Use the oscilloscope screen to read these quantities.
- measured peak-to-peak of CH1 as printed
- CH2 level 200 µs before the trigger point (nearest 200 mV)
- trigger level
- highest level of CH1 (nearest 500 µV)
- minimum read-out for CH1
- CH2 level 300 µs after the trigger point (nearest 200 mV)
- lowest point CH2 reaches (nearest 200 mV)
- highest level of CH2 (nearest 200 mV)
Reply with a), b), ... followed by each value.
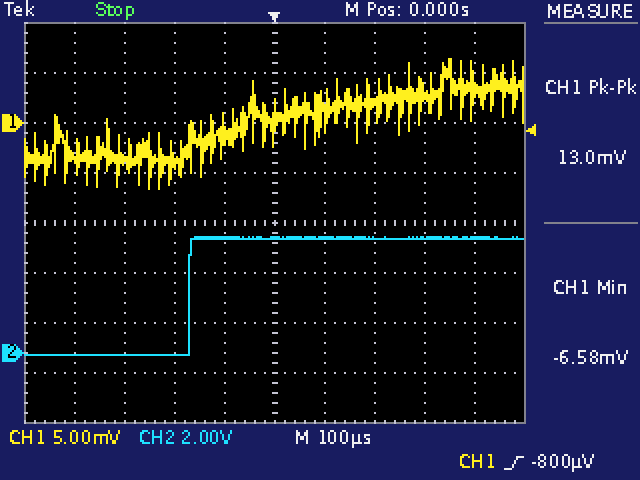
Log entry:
a) 13.0 mV
b) 0.0 V
c) -800 µV
d) 6.5 mV
e) -6.58 mV
f) 4.6 V
g) 0.0 V
h) 4.6 V
